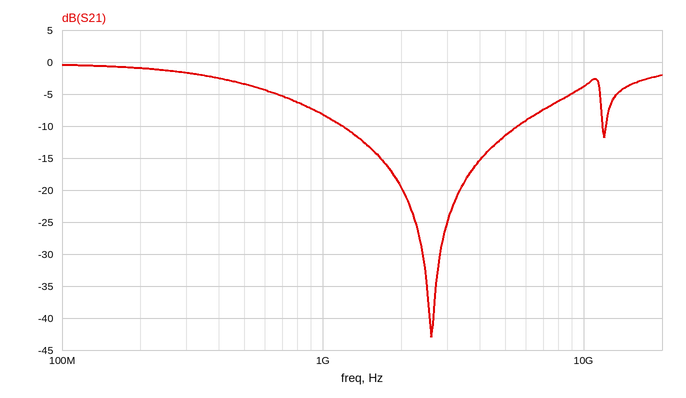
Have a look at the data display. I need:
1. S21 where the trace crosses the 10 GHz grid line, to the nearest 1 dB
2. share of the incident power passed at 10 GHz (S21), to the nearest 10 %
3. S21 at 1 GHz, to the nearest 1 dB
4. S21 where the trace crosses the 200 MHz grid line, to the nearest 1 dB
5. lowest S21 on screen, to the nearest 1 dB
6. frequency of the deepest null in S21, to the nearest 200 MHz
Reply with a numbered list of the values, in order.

1. -4 dB
2. 40 %
3. -8 dB
4. -1 dB
5. -43 dB
6. 2.6 GHz
